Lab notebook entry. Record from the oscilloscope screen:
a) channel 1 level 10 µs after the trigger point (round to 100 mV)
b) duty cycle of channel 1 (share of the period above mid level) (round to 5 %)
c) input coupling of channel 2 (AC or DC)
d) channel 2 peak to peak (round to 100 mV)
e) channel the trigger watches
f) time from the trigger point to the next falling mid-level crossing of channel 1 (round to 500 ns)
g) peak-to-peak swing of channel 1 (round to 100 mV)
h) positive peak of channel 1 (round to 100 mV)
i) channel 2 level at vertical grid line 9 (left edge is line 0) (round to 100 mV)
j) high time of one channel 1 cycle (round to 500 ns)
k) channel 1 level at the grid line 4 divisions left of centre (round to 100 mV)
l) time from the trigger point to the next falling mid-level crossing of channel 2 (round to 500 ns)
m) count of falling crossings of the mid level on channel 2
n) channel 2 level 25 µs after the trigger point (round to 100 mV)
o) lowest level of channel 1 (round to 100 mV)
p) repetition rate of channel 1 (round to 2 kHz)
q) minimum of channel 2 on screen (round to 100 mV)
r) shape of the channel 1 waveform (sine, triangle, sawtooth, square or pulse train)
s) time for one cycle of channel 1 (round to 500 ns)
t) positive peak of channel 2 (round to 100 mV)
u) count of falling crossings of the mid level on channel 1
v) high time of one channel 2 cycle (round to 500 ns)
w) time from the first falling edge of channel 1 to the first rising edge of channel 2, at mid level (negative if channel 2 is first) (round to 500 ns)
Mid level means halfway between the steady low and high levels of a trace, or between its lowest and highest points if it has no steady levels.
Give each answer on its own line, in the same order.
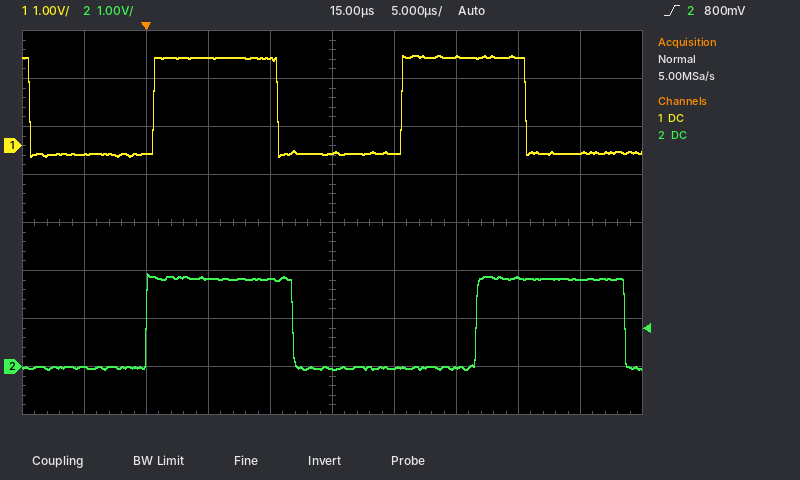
1.8 V
50 %
DC
2.0 V
channel 2
10.5 µs
2.1 V
1.9 V
1.8 V
10.0 µs
-200 mV
12.0 µs
2
0.0 V
-200 mV
50 kHz
-100 mV
square
20.0 µs
1.9 V
3
12.0 µs
+9.5 µs
